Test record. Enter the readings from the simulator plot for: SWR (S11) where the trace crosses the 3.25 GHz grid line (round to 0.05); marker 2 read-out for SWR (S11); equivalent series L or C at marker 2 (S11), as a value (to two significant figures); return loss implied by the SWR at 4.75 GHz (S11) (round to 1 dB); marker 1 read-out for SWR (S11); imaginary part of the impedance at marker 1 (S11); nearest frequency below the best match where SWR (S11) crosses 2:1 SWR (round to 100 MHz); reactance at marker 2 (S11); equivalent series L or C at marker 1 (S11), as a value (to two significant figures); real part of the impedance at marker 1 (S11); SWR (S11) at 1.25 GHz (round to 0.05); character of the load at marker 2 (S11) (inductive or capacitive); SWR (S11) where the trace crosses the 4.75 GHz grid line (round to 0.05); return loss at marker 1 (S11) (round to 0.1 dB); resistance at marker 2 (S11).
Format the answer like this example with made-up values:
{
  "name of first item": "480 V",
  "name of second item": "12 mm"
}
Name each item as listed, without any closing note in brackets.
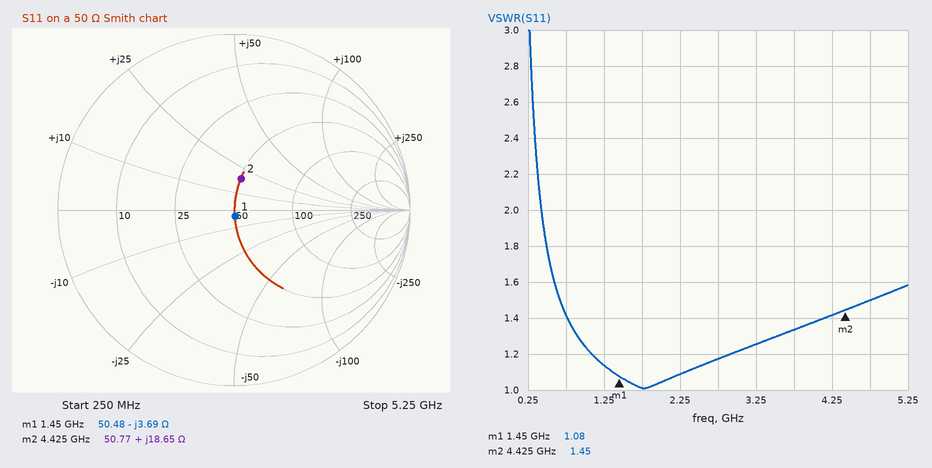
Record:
{
  "SWR (S11) where the trace crosses the 3.25 GHz grid line": "1.25",
  "marker 2 read-out for SWR": "1.45",
  "equivalent series L or C at marker 2 (S11), as a value": "670 pH",
  "return loss implied by the SWR at 4.75 GHz (S11)": "14 dB",
  "marker 1 read-out for SWR": "1.08",
  "imaginary part of the impedance at marker 1": "-3.69 Ω",
  "nearest frequency below the best match where SWR (S11) crosses 2:1 SWR": "400 MHz",
  "reactance at marker 2": "+18.65 Ω",
  "equivalent series L or C at marker 1 (S11), as a value": "30 pF",
  "real part of the impedance at marker 1": "50.48 Ω",
  "SWR (S11) at 1.25 GHz": "1.15",
  "character of the load at marker 2 (S11)": "inductive",
  "SWR (S11) where the trace crosses the 4.75 GHz grid line": "1.50",
  "return loss at marker 1 (S11)": "28.6 dB",
  "resistance at marker 2": "50.77 Ω"
}
